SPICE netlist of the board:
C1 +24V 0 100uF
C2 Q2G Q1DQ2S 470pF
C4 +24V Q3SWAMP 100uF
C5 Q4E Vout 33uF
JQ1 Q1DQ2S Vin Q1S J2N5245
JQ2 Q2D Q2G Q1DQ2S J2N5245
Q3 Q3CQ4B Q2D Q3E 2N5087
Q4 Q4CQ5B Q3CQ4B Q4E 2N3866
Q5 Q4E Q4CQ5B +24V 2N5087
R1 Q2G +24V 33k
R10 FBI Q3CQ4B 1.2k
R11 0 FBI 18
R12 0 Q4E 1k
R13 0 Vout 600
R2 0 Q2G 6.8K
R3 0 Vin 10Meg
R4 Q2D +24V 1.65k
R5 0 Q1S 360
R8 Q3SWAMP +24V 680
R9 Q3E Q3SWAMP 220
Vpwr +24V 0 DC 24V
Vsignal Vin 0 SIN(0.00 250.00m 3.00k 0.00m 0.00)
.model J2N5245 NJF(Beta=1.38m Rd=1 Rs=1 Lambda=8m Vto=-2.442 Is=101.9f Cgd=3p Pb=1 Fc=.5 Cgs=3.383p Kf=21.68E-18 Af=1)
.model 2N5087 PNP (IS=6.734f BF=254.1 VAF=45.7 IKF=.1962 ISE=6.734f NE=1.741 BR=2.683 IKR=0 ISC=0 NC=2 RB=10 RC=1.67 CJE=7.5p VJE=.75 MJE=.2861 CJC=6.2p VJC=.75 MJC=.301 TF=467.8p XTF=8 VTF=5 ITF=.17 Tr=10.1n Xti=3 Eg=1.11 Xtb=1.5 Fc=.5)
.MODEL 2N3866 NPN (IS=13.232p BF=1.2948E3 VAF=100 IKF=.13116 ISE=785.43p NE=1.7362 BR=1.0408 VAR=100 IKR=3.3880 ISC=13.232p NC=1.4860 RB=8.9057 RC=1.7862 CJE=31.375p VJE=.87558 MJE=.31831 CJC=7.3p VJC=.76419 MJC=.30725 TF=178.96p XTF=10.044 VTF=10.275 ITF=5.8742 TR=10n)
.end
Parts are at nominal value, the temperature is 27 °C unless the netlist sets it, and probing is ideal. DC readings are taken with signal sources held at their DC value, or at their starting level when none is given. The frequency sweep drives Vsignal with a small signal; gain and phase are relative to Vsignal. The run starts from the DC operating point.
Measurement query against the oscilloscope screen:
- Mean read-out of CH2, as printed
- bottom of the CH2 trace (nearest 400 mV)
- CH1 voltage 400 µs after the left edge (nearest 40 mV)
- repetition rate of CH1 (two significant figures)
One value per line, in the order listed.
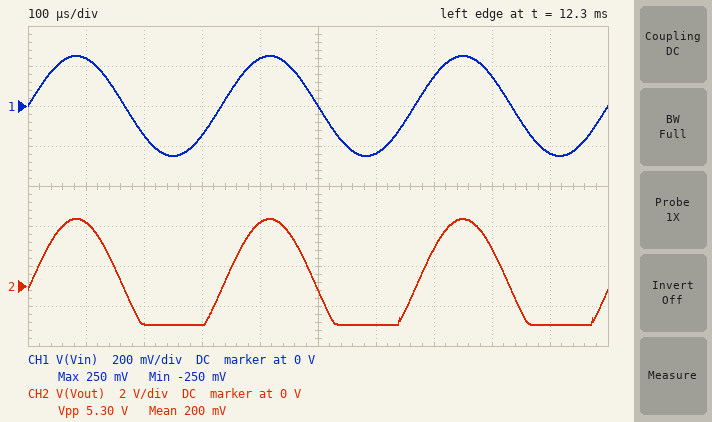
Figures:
200 mV
-2.0 V
240 mV
3.0 kHz
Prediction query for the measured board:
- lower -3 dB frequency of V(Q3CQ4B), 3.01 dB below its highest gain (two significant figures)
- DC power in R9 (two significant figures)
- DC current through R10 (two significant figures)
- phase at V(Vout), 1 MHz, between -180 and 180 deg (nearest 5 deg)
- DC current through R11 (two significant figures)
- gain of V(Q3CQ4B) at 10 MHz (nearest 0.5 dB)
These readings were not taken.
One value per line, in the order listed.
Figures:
8.6 Hz
4.3 mW
4.4 mA
-55 deg
4.4 mA
-3.0 dB
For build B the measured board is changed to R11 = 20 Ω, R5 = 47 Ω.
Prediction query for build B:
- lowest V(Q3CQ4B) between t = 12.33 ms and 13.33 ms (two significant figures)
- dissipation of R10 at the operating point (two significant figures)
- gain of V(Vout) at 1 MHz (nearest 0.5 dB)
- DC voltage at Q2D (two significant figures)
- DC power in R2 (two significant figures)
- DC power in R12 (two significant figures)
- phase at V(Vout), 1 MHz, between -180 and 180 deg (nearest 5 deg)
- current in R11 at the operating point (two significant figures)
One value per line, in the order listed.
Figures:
4.7 V
140 mW
29.0 dB
13 V
2.5 mW
170 mW
-60 deg
11 mA
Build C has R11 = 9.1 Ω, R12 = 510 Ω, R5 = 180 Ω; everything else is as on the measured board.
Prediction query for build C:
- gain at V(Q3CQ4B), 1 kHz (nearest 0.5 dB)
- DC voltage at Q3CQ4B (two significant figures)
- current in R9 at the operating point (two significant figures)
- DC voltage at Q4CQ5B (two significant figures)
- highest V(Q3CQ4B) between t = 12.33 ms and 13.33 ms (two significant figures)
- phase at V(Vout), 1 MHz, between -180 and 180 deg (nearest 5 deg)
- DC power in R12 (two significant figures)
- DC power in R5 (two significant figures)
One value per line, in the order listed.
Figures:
27.0 dB
8.1 V
6.7 mA
23 V
14 V
-50 deg
120 mW
3.0 mW
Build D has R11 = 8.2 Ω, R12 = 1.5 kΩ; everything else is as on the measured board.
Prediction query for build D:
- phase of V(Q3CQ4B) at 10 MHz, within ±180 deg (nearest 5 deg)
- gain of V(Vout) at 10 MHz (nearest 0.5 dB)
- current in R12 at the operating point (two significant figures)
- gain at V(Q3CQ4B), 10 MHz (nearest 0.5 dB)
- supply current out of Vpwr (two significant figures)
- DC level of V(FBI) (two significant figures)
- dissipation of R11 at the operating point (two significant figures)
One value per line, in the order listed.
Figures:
-120 deg
-7.5 dB
3.3 mA
-6.0 dB
11 mA
36 mV
160 µW
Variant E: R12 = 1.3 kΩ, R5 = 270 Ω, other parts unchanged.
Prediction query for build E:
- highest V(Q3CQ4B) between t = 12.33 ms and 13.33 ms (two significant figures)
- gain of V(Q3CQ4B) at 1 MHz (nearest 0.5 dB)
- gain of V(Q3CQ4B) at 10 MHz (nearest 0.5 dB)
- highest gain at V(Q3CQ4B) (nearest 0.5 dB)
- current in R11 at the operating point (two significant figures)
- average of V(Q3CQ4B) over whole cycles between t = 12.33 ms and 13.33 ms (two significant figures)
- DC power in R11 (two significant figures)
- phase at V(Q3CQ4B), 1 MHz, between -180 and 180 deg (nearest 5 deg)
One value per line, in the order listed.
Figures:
11 V
22.5 dB
-1.5 dB
24.5 dB
5.3 mA
6.5 V
510 µW
-50 deg
